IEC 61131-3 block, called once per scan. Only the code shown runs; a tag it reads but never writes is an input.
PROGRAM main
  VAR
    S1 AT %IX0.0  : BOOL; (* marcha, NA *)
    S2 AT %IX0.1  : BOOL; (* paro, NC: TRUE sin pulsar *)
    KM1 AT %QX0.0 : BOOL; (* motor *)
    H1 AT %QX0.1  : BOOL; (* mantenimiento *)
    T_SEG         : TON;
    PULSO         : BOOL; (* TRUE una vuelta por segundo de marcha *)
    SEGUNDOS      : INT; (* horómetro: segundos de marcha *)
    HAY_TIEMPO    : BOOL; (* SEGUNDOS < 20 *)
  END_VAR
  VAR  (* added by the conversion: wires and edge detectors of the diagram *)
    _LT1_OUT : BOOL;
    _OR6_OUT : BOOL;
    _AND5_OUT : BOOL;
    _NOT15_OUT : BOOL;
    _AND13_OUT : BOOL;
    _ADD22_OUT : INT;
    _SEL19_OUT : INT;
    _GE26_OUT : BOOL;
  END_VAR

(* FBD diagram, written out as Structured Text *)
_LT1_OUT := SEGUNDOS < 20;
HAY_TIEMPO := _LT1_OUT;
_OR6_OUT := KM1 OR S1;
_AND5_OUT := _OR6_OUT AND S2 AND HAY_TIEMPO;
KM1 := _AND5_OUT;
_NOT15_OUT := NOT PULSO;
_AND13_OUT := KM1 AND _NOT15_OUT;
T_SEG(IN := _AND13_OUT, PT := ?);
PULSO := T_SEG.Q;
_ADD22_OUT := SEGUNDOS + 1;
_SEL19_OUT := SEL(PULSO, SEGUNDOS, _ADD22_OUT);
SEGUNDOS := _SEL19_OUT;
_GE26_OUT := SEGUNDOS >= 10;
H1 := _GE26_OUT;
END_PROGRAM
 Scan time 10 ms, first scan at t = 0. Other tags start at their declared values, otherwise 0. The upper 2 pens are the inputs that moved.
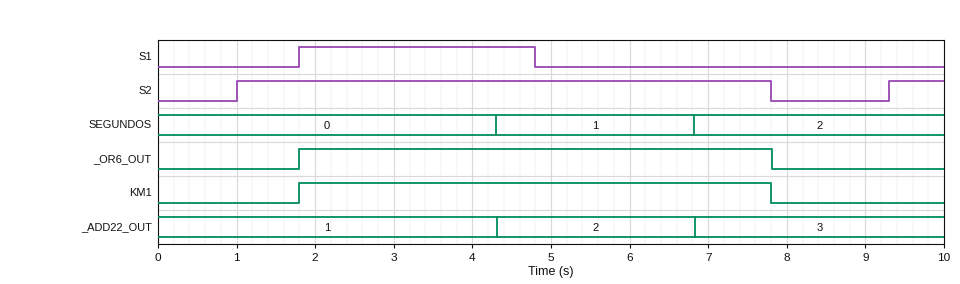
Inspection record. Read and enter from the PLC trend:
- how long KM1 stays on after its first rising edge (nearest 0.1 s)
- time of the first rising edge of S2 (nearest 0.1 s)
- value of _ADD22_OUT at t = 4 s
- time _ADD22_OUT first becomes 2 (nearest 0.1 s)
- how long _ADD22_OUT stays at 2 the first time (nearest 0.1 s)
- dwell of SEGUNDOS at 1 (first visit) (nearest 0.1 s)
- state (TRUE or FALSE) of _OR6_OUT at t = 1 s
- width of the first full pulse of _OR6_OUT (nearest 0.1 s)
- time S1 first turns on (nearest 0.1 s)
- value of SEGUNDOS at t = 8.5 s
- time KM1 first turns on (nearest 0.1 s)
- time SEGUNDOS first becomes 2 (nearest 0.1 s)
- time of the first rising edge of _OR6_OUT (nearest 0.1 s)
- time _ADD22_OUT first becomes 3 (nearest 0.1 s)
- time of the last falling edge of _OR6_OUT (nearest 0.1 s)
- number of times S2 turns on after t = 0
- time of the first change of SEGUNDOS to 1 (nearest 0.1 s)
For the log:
6.0 s
1.0 s
1
4.3 s
2.5 s
2.5 s
FALSE
6.0 s
1.8 s
2
1.8 s
6.8 s
1.8 s
6.8 s
7.8 s
2
4.3 s
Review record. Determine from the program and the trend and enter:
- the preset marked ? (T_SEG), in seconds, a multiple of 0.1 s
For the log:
2.5 s
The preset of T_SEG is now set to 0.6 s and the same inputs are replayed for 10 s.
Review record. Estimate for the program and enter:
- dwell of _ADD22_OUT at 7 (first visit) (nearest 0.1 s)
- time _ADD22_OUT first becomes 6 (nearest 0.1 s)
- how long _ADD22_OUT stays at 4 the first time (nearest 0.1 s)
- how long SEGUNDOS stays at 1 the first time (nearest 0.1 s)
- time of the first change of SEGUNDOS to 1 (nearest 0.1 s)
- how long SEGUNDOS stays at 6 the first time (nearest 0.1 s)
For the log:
0.6 s
4.9 s
0.6 s
0.6 s
2.4 s
0.6 s
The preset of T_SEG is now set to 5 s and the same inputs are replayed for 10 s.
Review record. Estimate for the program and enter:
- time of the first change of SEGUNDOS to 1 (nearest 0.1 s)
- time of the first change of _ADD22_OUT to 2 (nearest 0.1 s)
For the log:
6.8 s
6.8 s
